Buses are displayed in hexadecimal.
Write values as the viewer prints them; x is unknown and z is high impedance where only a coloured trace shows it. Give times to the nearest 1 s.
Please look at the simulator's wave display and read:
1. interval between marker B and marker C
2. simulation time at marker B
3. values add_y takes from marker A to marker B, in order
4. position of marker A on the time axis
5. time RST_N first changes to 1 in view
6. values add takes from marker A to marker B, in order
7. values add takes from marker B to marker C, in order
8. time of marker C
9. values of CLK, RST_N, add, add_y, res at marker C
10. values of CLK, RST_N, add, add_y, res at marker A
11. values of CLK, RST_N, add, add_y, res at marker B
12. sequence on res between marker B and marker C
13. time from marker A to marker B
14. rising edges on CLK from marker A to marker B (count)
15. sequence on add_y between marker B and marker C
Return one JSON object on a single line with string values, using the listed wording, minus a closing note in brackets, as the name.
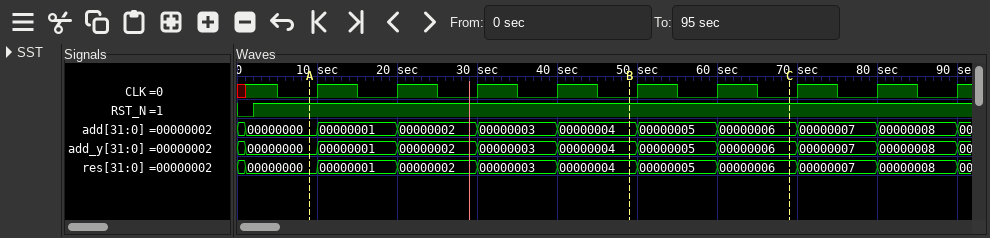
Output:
{"interval between marker B and marker C": "20 s", "simulation time at marker B": "49 s", "values add_y takes from marker A to marker B, in order": "00000000, 00000001, 00000002, 00000003, 00000004", "position of marker A on the time axis": "9 s", "time RST_N first changes to 1 in view": "2 s", "values add takes from marker A to marker B, in order": "00000000, 00000001, 00000002, 00000003, 00000004", "values add takes from marker B to marker C, in order": "00000004, 00000005, 00000006", "time of marker C": "69 s", "values of CLK, RST_N, add, add_y, res at marker C": "CLK=0, RST_N=1, add=00000006, add_y=00000006, res=00000006", "values of CLK, RST_N, add, add_y, res at marker A": "CLK=0, RST_N=1, add=00000000, add_y=00000000, res=00000000", "values of CLK, RST_N, add, add_y, res at marker B": "CLK=0, RST_N=1, add=00000004, add_y=00000004, res=00000004", "sequence on res between marker B and marker C": "00000004, 00000005, 00000006", "time from marker A to marker B": "40 s", "rising edges on CLK from marker A to marker B": "4", "sequence on add_y between marker B and marker C": "00000004, 00000005, 00000006"}
